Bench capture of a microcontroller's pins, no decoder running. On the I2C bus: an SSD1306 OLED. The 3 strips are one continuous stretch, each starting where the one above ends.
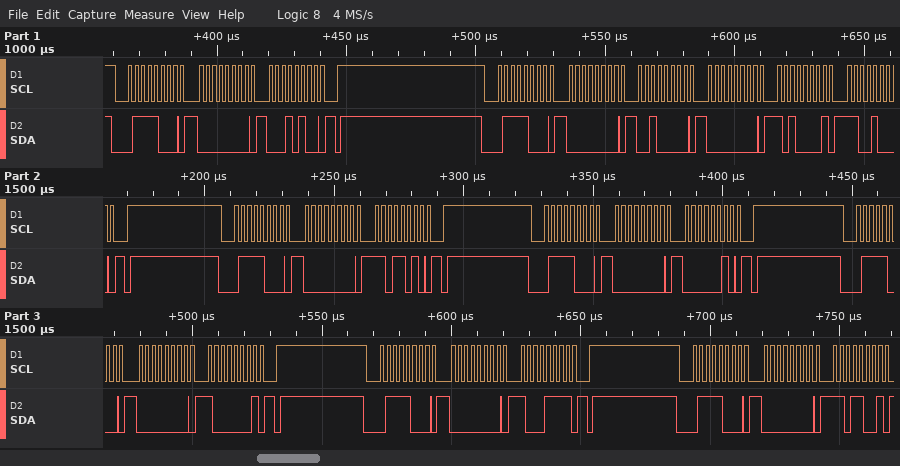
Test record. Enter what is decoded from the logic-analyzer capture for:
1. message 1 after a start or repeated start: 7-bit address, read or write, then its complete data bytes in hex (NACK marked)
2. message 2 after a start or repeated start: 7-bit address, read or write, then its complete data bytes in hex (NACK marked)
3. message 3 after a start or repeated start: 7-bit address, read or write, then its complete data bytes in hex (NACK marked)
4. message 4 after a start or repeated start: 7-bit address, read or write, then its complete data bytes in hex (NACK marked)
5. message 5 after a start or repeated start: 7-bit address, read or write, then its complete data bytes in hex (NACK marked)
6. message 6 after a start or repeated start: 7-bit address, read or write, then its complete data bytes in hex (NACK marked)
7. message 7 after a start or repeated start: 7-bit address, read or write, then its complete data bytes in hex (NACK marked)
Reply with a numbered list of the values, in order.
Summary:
1. 0x3C write: 00 14
2. 0x3C write: 00 20 00 A1 C8
3. 0x3C write: 00 DA
4. 0x3C write: 00 02
5. 0x3C write: 00 81
6. 0x3C write: 00 8F
7. 0x3C write: 00 D9
